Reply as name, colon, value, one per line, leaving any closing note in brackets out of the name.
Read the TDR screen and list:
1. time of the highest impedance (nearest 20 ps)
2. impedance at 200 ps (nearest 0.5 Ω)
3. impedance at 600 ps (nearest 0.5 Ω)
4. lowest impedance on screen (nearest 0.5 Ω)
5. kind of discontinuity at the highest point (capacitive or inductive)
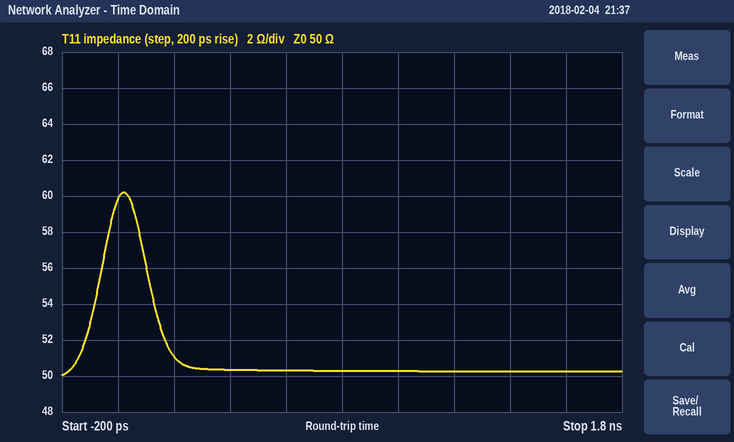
time of the highest impedance: 20 ps
impedance at 200 ps: 51.0 Ω
impedance at 600 ps: 50.5 Ω
lowest impedance on screen: 50.0 Ω
kind of discontinuity at the highest point: inductive
